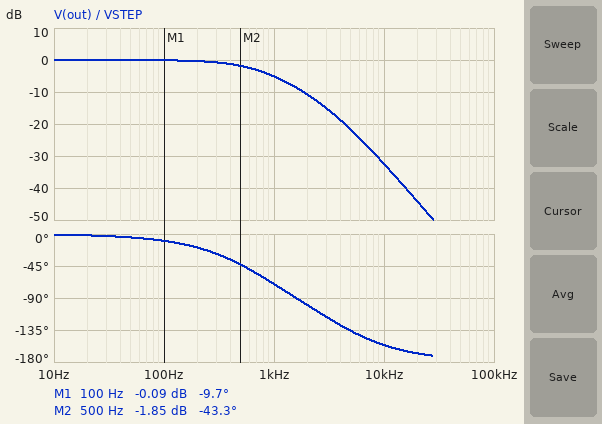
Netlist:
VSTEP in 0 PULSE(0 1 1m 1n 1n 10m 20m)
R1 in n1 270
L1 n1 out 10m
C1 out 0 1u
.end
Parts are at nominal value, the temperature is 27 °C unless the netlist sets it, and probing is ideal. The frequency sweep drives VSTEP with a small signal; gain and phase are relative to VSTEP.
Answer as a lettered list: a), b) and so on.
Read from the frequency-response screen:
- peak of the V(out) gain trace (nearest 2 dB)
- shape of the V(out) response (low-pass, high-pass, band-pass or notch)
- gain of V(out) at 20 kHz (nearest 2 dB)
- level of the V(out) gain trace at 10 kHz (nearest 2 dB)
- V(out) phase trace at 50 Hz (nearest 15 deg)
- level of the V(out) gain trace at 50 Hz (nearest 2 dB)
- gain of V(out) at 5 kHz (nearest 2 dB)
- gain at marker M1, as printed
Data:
a) 0 dB
b) low-pass
c) -44 dB
d) -32 dB
e) 0 deg
f) 0 dB
g) -22 dB
h) -0.09 dB
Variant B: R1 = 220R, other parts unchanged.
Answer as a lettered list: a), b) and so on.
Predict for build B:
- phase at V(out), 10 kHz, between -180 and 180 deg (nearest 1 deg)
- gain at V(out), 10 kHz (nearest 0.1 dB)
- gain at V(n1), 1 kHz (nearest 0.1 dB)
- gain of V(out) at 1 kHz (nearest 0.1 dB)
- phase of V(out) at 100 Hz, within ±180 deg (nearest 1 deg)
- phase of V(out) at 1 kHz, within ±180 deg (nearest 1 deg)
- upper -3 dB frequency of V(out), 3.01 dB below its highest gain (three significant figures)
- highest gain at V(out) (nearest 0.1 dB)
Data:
a) -160 deg
b) -32.2 dB
c) -7.9 dB
d) -3.6 dB
e) -8 deg
f) -66 deg
g) 896 Hz
h) 0 dB
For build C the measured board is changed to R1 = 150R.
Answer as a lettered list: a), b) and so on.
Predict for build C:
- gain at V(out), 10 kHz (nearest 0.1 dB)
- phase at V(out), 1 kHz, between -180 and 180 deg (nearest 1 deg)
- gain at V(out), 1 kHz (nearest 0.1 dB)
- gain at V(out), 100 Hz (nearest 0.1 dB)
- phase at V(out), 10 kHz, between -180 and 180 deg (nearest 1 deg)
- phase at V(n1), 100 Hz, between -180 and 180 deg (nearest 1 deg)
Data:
a) -32.0 dB
b) -57 deg
c) -1.0 dB
d) 0 dB
e) -166 deg
f) -5 deg
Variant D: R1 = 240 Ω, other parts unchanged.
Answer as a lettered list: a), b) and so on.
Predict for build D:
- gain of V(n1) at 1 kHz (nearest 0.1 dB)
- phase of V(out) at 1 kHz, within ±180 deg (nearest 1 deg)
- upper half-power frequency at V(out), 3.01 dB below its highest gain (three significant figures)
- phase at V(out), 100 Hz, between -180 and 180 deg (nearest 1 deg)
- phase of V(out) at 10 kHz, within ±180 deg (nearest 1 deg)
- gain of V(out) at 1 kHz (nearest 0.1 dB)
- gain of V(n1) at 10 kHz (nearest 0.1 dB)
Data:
a) -8.6 dB
b) -68 deg
c) 795 Hz
d) -9 deg
e) -159 deg
f) -4.2 dB
g) -0.6 dB
